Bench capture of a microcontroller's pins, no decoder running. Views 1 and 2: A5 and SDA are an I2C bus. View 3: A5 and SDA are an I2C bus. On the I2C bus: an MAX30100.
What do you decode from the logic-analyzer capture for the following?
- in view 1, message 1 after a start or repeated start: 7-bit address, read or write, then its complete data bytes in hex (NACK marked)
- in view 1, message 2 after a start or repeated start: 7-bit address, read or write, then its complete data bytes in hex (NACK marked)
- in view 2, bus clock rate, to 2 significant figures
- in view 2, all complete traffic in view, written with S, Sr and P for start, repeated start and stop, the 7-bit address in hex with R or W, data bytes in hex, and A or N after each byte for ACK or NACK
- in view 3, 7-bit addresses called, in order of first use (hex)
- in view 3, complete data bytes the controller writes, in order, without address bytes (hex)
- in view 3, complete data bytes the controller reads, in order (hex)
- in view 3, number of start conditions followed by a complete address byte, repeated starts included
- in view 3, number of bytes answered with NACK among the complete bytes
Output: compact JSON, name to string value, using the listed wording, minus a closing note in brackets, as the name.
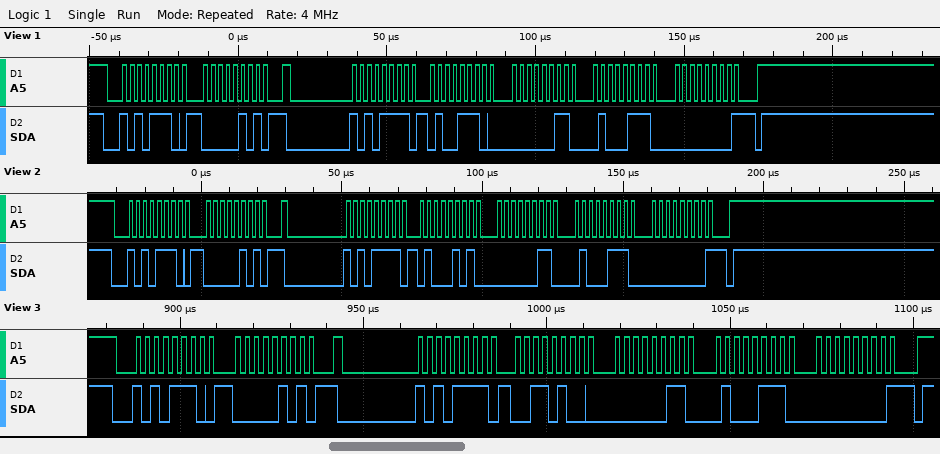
{"in view 1, message 1 after a start or repeated start: 7-bit address, read or write, then its complete data bytes in hex": "0x57 write: 05", "in view 1, message 2 after a start or repeated start: 7-bit address, read or write, then its complete data bytes in hex": "0x57 read: 4E 03 47 00 NACK", "in view 2, bus clock rate, to 2 significant figures": "400 kHz", "in view 2, all complete traffic in view, written with S, Sr and P for start, repeated start and stop, the 7-bit address in hex with R or W, data bytes in hex, and A or N after each byte for ACK or NACK": "S 57W A 05 A Sr 57R A 45 A 03 A 47 A 00 N P", "in view 3, 7-bit addresses called, in order of first use": "0x57", "in view 3, complete data bytes the controller writes, in order, without address bytes": "05", "in view 3, complete data bytes the controller reads, in order": "34 03 47 00", "in view 3, number of start conditions followed by a complete address byte, repeated starts included": "2", "in view 3, number of bytes answered with NACK among the complete bytes": "1"}
